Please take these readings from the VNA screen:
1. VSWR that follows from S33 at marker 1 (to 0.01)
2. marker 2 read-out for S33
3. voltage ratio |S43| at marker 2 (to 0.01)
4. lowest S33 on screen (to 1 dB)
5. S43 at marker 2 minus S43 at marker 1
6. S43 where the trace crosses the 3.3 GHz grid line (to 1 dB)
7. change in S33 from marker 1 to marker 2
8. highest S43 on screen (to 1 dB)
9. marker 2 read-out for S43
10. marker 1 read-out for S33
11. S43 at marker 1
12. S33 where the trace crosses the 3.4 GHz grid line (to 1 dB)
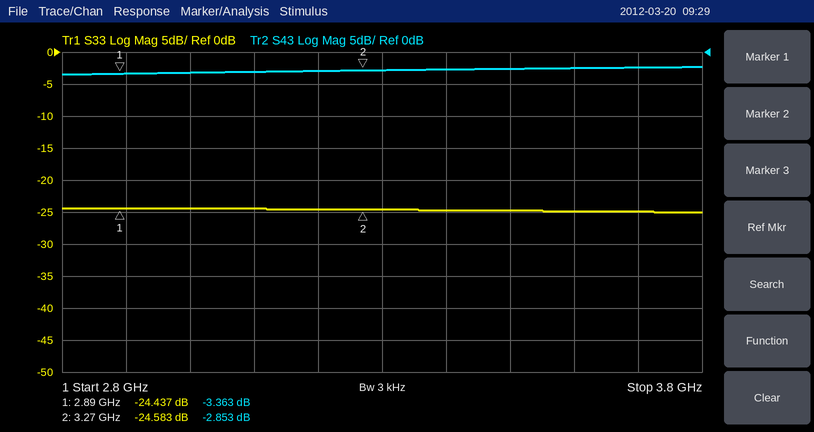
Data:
1.13
-24.583 dB
0.72
-25 dB
0.510 dB
-3 dB
-0.146 dB
-2 dB
-2.853 dB
-24.437 dB
-3.363 dB
-25 dB
